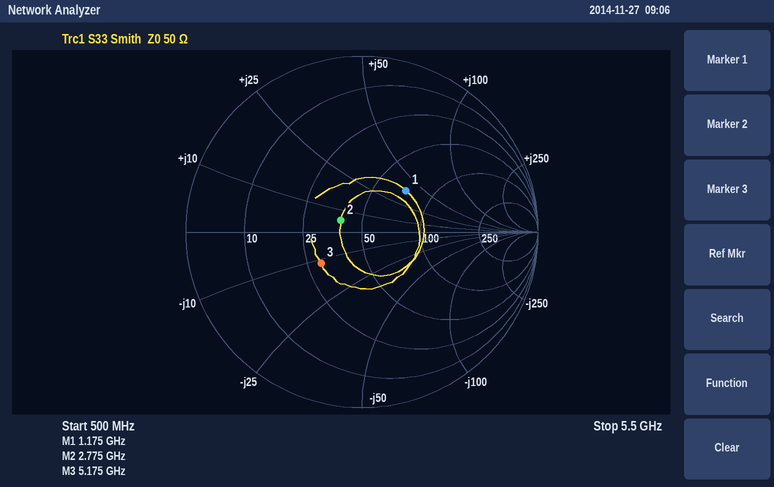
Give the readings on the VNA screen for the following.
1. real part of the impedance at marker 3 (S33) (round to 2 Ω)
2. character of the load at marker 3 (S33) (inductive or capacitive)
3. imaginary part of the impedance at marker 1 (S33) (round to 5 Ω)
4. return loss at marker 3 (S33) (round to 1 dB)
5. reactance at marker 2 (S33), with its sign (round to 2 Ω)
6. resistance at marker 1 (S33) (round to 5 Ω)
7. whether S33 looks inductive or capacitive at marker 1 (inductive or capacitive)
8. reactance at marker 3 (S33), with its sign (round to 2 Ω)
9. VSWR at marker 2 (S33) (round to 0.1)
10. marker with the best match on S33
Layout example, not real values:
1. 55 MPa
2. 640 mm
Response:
1. 30 Ω
2. capacitive
3. +40 Ω
4. 11 dB
5. +6 Ω
6. 70 Ω
7. inductive
8. -12 Ω
9. 1.3
10. marker 2
